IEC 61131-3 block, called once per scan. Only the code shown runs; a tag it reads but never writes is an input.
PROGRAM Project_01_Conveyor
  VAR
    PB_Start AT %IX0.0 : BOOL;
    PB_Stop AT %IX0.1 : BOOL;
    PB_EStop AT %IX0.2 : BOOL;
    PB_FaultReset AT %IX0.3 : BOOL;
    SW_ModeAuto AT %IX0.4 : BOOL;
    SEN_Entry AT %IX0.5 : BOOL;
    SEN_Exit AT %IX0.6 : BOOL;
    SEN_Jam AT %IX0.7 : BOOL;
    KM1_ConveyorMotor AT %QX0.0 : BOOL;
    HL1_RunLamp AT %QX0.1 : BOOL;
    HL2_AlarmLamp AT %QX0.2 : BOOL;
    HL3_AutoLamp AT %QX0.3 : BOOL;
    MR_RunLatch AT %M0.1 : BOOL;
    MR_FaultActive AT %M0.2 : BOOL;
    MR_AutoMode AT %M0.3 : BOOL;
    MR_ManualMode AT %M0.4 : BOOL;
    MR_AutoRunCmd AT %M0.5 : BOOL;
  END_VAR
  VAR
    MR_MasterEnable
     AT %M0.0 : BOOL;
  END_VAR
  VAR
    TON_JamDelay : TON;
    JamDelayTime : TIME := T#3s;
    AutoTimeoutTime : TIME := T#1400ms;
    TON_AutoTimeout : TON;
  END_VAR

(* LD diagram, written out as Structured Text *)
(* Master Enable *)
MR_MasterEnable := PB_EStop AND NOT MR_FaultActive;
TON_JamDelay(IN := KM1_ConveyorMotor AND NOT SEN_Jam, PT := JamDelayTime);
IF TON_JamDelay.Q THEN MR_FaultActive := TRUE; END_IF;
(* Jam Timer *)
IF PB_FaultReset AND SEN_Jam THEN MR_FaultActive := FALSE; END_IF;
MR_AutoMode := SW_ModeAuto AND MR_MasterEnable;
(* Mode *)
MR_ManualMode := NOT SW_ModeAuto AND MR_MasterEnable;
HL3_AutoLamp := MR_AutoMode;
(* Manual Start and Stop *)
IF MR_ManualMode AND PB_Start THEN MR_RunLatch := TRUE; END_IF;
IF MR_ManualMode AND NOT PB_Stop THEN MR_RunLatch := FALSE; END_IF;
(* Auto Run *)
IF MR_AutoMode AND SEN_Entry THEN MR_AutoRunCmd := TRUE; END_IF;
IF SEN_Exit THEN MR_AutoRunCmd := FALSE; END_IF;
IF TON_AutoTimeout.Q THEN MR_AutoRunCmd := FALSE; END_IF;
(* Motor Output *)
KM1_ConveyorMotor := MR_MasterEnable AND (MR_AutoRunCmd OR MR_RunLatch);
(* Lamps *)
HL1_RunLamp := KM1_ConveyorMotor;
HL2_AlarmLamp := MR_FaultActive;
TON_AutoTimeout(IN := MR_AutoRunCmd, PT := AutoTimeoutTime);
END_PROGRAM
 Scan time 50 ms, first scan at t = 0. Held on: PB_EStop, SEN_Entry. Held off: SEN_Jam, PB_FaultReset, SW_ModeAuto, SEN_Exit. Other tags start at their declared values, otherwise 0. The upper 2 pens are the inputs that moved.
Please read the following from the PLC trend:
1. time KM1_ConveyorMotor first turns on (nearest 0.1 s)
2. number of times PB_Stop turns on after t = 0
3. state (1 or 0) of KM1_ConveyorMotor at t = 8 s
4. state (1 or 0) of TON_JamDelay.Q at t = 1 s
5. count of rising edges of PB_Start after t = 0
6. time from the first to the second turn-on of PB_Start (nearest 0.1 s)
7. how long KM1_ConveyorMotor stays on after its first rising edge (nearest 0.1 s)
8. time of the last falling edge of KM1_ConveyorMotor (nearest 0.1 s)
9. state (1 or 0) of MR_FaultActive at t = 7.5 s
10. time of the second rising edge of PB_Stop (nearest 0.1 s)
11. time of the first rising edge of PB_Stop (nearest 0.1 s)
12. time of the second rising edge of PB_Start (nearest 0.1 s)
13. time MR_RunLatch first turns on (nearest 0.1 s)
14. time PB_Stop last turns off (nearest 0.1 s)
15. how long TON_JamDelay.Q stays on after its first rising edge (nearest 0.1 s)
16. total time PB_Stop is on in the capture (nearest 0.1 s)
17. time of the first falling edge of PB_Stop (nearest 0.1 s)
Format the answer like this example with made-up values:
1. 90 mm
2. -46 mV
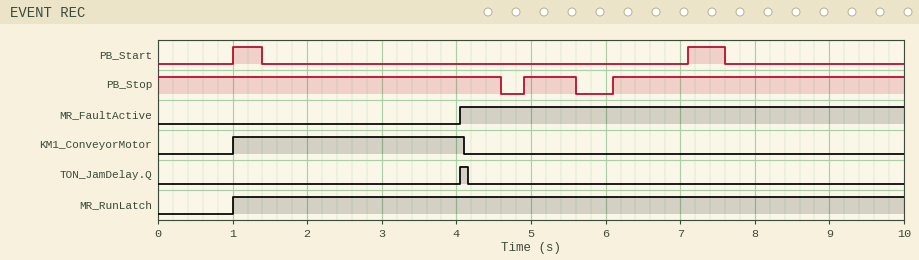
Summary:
1. 1.0 s
2. 2
3. 0
4. 0
5. 2
6. 6.1 s
7. 3.1 s
8. 4.1 s
9. 1
10. 6.1 s
11. 4.9 s
12. 7.1 s
13. 1.0 s
14. 5.6 s
15. 0.1 s
16. 9.2 s
17. 4.6 s
